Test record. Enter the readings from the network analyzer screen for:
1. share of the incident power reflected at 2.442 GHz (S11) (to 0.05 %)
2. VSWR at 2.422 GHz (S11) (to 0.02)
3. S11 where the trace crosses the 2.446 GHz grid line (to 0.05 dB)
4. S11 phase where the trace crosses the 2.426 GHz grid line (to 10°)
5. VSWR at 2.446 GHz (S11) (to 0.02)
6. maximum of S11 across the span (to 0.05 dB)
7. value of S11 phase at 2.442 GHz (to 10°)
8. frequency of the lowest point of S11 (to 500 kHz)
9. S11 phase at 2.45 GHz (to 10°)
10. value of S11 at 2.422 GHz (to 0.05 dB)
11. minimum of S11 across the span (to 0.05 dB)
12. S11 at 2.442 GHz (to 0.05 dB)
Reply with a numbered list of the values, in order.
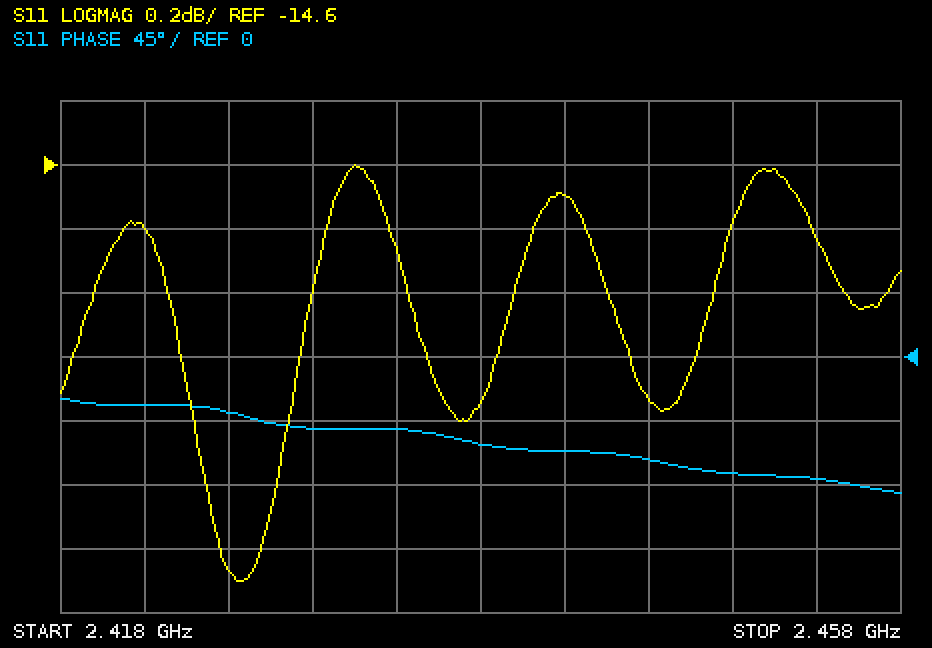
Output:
1. 3.40 %
2. 1.44
3. -15.35 dB
4. -40°
5. 1.42
6. -14.60 dB
7. -70°
8. 2.4265 GHz
9. -80°
10. -14.80 dB
11. -15.90 dB
12. -14.70 dB
